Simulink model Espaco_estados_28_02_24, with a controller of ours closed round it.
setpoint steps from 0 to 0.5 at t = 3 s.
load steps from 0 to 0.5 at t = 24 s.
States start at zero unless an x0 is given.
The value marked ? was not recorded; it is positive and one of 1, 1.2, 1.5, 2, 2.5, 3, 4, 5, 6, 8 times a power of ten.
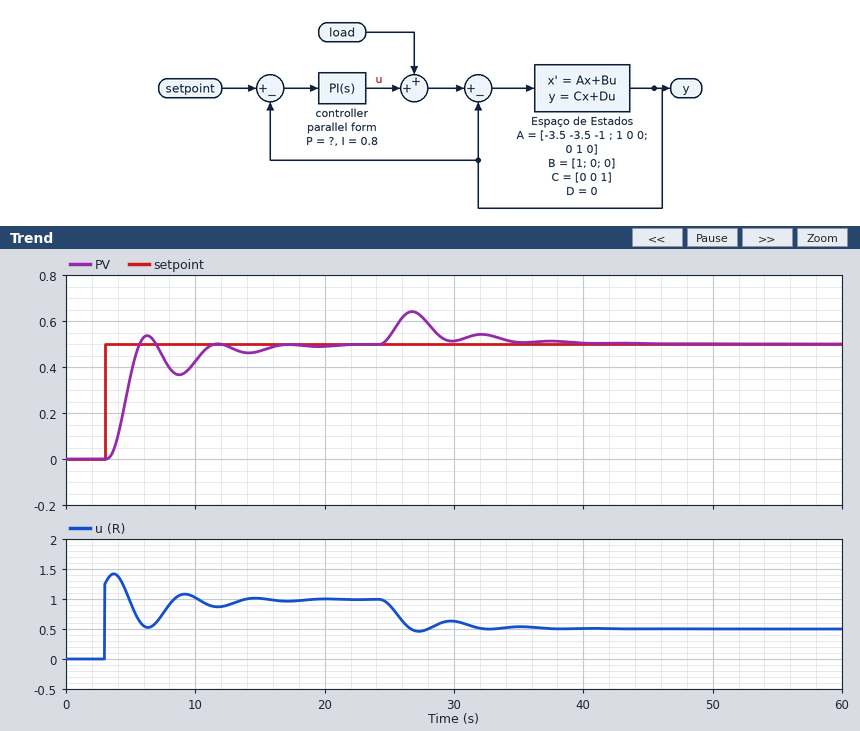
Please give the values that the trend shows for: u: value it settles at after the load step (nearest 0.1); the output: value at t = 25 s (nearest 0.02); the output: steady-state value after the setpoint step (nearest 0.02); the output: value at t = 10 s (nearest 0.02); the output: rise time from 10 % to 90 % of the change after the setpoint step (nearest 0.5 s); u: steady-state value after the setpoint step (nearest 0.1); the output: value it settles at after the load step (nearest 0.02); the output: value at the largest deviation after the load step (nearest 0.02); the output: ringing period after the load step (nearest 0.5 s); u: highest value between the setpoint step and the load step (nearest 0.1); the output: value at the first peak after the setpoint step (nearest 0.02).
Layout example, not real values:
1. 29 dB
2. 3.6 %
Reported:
1. 0.5
2. 0.54
3. 0.50
4. 0.42
5. 1.5 s
6. 1.0
7. 0.50
8. 0.64
9. 5.5 s
10. 1.4
11. 0.54
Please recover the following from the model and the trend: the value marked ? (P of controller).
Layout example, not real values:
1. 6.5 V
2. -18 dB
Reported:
1. 2.5
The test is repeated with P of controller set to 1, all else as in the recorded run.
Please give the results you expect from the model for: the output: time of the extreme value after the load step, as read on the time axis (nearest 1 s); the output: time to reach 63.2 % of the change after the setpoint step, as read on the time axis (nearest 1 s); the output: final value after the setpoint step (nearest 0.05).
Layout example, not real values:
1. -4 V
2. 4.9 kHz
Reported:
1. 27 s
2. 6 s
3. 0.50
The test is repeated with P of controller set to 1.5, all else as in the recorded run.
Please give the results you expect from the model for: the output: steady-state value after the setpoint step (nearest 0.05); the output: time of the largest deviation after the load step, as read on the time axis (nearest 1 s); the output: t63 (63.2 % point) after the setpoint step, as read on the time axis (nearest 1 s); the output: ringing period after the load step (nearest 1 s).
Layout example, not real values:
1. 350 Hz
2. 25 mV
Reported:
1. 0.50
2. 27 s
3. 5 s
4. 6 s
